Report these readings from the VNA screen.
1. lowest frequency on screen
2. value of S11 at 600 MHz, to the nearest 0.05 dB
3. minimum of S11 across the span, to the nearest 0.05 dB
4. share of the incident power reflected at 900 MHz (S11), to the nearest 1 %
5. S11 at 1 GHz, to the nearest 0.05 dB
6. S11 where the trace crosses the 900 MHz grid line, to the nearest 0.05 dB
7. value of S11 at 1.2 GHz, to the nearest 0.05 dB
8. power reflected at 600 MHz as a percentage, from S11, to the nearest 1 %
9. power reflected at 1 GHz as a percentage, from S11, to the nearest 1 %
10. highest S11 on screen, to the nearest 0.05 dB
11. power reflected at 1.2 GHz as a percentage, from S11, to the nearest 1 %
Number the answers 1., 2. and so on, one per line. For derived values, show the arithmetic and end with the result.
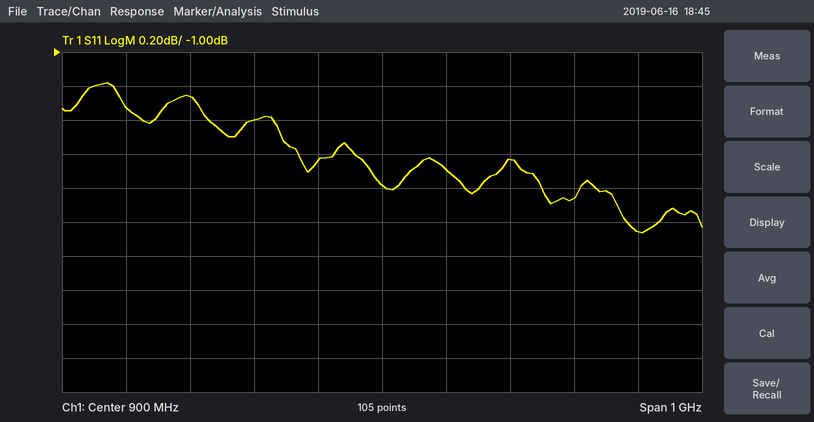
1. 400 MHz
2. -1.25 dB
3. -2.05 dB
4. 10^(-1.8/10) ≈ 66 %
5. -1.70 dB
6. -1.80 dB
7. -1.85 dB
8. 10^(-1.25/10) ≈ 75 %
9. 10^(-1.7/10) ≈ 68 %
10. -1.20 dB
11. 10^(-1.85/10) ≈ 65 %
